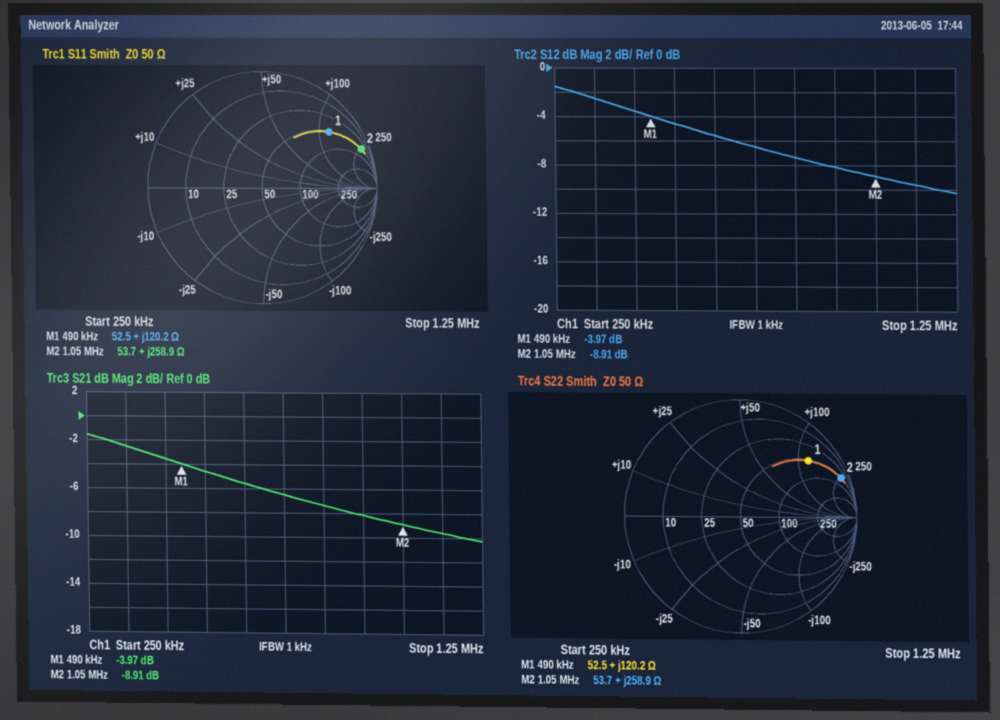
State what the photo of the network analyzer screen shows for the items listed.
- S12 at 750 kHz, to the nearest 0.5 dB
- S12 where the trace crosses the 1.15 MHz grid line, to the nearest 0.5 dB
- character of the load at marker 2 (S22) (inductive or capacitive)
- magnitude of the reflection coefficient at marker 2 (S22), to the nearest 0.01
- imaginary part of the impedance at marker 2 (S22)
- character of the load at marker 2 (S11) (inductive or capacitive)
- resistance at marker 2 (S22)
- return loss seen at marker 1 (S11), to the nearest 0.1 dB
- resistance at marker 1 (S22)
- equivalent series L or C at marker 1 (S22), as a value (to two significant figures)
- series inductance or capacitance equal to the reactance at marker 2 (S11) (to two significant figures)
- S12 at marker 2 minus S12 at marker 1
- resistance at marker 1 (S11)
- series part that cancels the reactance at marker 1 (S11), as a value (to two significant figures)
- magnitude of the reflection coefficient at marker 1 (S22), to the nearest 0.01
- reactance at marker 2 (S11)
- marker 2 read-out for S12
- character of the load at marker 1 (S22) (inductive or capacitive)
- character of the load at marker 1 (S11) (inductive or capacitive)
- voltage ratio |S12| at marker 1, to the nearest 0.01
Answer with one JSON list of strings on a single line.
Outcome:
["-6.5 dB", "-9.5 dB", "inductive", "0.93", "+258.9 Ω", "inductive", "53.7 Ω", "2.4 dB", "52.5 Ω", "39 µH", "39 µH", "-4.94 dB", "52.5 Ω", "2.7 nF", "0.76", "+258.9 Ω", "-8.91 dB", "inductive", "inductive", "0.63"]
